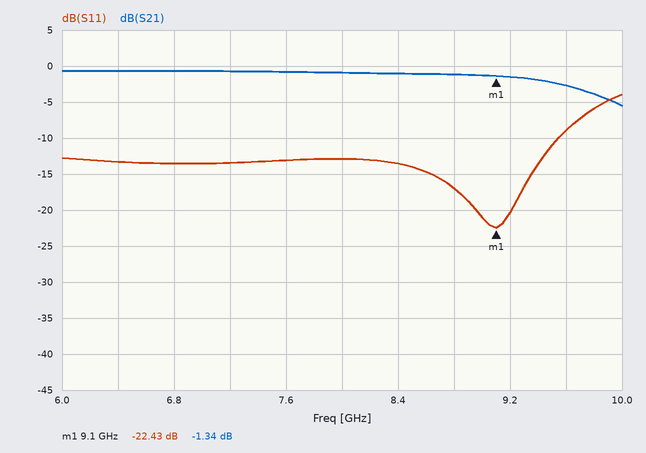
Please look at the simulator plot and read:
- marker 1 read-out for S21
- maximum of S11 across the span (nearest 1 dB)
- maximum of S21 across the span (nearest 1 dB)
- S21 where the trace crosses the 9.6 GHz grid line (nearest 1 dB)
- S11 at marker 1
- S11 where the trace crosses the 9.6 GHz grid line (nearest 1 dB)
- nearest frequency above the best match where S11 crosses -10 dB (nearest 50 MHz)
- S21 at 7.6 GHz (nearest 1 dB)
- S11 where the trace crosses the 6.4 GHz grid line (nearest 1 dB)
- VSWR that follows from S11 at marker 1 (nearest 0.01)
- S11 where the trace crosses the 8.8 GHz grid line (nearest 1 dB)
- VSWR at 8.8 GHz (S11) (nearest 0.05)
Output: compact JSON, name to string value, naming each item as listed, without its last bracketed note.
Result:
{"marker 1 read-out for S21": "-1.34 dB", "maximum of S11 across the span": "-4 dB", "maximum of S21 across the span": "-1 dB", "S21 where the trace crosses the 9.6 GHz grid line": "-3 dB", "S11 at marker 1": "-22.43 dB", "S11 where the trace crosses the 9.6 GHz grid line": "-9 dB", "nearest frequency above the best match where S11 crosses -10 dB": "9.55 GHz", "S21 at 7.6 GHz": "-1 dB", "S11 where the trace crosses the 6.4 GHz grid line": "-13 dB", "VSWR that follows from S11 at marker 1": "1.16", "S11 where the trace crosses the 8.8 GHz grid line": "-17 dB", "VSWR at 8.8 GHz (S11)": "1.35"}
